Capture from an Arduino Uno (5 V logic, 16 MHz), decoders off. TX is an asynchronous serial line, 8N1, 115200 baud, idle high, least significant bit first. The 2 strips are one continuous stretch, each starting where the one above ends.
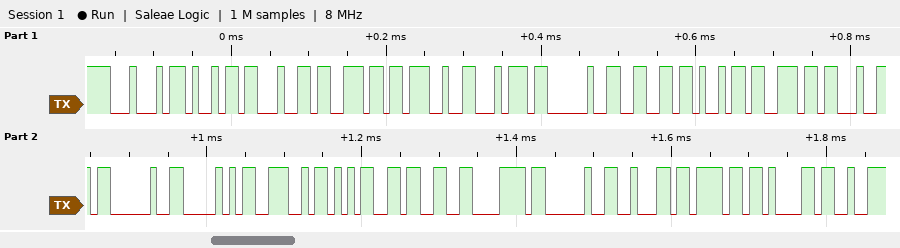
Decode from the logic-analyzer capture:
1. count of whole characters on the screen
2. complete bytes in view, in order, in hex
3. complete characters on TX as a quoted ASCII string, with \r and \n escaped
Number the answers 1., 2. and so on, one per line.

1. 21
2. 44 69 64 6E 27 74 20 66 69 6E 64 20 50 4E 35 33 78 20 62 6F 61
3. "Didn't find PN53x boa"
